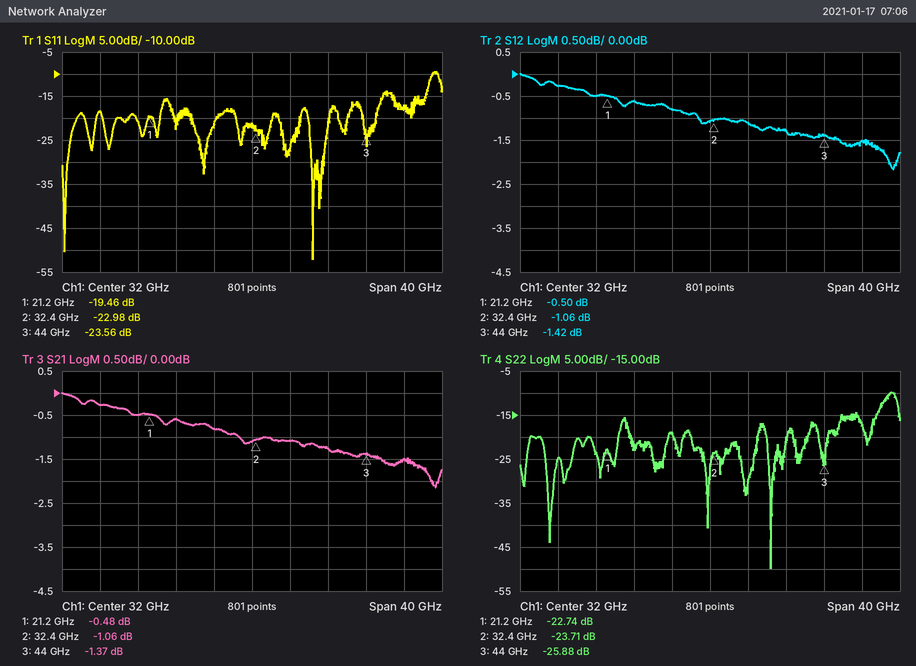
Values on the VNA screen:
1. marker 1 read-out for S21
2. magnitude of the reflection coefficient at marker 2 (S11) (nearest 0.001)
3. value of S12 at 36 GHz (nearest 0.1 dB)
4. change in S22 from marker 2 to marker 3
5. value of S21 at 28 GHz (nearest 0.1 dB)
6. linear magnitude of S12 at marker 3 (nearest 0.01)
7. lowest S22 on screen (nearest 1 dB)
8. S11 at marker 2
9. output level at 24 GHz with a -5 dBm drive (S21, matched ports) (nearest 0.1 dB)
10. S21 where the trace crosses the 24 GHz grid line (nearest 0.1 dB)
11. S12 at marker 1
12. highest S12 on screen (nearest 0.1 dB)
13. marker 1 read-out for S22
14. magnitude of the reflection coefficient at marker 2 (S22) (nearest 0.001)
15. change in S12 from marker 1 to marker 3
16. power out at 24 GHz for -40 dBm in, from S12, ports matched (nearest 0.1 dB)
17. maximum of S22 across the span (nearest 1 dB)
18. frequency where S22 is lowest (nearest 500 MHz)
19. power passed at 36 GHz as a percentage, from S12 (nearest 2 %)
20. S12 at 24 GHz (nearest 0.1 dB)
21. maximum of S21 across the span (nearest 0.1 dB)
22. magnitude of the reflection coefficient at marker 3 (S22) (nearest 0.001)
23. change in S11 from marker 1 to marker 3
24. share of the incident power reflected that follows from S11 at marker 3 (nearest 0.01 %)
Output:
-0.48 dB
0.071
-1.1 dB
-2.17 dB
-0.8 dB
0.85
-50 dB
-22.98 dB
-5.6 dBm
-0.6 dB
-0.50 dB
0.0 dB
-22.74 dB
0.065
-0.92 dB
-40.6 dBm
-10 dB
38.5 GHz
78 %
-0.6 dB
0.0 dB
0.051
-4.10 dB
0.44 %
